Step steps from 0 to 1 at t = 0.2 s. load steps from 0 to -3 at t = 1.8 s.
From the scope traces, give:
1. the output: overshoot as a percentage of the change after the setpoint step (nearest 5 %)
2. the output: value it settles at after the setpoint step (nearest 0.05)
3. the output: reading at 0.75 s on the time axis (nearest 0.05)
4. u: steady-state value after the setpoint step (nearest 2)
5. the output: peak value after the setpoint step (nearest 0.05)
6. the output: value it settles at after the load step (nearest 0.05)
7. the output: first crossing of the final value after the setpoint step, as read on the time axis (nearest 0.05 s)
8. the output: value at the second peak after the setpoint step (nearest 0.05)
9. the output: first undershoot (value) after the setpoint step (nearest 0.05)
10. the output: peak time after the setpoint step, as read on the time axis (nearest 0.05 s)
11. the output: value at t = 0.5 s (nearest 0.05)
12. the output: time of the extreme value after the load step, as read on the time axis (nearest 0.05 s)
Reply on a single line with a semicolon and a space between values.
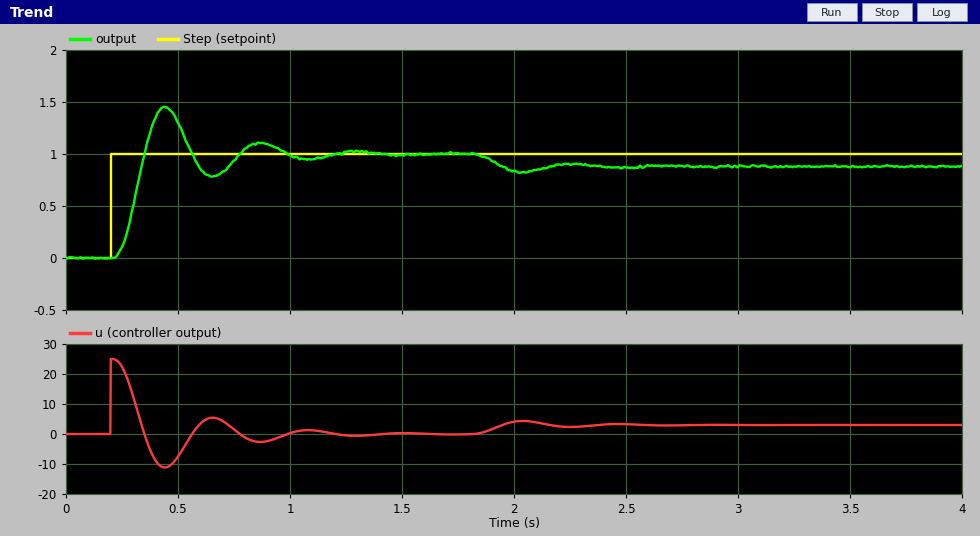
45 %; 1.00; 0.95; 0; 1.45; 0.90; 0.35 s; 1.10; 0.80; 0.45 s; 1.30; 2.05 s
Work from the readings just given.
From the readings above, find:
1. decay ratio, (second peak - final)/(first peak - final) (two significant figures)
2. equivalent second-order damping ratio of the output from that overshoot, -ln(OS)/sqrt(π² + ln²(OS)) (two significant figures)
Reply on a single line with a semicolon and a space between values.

0.22; 0.25
